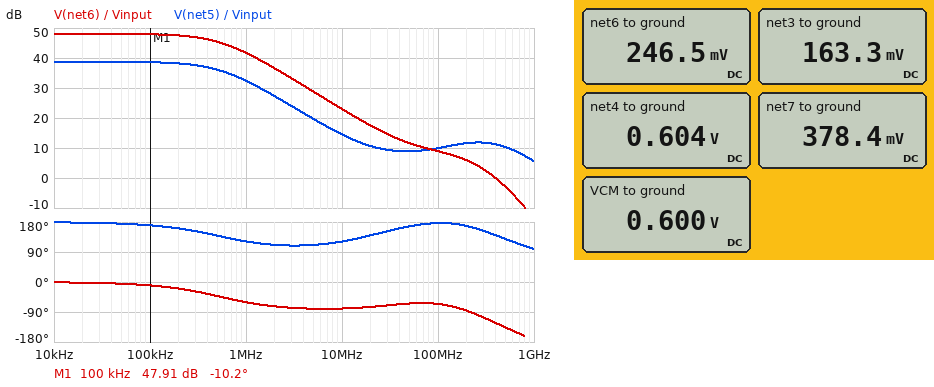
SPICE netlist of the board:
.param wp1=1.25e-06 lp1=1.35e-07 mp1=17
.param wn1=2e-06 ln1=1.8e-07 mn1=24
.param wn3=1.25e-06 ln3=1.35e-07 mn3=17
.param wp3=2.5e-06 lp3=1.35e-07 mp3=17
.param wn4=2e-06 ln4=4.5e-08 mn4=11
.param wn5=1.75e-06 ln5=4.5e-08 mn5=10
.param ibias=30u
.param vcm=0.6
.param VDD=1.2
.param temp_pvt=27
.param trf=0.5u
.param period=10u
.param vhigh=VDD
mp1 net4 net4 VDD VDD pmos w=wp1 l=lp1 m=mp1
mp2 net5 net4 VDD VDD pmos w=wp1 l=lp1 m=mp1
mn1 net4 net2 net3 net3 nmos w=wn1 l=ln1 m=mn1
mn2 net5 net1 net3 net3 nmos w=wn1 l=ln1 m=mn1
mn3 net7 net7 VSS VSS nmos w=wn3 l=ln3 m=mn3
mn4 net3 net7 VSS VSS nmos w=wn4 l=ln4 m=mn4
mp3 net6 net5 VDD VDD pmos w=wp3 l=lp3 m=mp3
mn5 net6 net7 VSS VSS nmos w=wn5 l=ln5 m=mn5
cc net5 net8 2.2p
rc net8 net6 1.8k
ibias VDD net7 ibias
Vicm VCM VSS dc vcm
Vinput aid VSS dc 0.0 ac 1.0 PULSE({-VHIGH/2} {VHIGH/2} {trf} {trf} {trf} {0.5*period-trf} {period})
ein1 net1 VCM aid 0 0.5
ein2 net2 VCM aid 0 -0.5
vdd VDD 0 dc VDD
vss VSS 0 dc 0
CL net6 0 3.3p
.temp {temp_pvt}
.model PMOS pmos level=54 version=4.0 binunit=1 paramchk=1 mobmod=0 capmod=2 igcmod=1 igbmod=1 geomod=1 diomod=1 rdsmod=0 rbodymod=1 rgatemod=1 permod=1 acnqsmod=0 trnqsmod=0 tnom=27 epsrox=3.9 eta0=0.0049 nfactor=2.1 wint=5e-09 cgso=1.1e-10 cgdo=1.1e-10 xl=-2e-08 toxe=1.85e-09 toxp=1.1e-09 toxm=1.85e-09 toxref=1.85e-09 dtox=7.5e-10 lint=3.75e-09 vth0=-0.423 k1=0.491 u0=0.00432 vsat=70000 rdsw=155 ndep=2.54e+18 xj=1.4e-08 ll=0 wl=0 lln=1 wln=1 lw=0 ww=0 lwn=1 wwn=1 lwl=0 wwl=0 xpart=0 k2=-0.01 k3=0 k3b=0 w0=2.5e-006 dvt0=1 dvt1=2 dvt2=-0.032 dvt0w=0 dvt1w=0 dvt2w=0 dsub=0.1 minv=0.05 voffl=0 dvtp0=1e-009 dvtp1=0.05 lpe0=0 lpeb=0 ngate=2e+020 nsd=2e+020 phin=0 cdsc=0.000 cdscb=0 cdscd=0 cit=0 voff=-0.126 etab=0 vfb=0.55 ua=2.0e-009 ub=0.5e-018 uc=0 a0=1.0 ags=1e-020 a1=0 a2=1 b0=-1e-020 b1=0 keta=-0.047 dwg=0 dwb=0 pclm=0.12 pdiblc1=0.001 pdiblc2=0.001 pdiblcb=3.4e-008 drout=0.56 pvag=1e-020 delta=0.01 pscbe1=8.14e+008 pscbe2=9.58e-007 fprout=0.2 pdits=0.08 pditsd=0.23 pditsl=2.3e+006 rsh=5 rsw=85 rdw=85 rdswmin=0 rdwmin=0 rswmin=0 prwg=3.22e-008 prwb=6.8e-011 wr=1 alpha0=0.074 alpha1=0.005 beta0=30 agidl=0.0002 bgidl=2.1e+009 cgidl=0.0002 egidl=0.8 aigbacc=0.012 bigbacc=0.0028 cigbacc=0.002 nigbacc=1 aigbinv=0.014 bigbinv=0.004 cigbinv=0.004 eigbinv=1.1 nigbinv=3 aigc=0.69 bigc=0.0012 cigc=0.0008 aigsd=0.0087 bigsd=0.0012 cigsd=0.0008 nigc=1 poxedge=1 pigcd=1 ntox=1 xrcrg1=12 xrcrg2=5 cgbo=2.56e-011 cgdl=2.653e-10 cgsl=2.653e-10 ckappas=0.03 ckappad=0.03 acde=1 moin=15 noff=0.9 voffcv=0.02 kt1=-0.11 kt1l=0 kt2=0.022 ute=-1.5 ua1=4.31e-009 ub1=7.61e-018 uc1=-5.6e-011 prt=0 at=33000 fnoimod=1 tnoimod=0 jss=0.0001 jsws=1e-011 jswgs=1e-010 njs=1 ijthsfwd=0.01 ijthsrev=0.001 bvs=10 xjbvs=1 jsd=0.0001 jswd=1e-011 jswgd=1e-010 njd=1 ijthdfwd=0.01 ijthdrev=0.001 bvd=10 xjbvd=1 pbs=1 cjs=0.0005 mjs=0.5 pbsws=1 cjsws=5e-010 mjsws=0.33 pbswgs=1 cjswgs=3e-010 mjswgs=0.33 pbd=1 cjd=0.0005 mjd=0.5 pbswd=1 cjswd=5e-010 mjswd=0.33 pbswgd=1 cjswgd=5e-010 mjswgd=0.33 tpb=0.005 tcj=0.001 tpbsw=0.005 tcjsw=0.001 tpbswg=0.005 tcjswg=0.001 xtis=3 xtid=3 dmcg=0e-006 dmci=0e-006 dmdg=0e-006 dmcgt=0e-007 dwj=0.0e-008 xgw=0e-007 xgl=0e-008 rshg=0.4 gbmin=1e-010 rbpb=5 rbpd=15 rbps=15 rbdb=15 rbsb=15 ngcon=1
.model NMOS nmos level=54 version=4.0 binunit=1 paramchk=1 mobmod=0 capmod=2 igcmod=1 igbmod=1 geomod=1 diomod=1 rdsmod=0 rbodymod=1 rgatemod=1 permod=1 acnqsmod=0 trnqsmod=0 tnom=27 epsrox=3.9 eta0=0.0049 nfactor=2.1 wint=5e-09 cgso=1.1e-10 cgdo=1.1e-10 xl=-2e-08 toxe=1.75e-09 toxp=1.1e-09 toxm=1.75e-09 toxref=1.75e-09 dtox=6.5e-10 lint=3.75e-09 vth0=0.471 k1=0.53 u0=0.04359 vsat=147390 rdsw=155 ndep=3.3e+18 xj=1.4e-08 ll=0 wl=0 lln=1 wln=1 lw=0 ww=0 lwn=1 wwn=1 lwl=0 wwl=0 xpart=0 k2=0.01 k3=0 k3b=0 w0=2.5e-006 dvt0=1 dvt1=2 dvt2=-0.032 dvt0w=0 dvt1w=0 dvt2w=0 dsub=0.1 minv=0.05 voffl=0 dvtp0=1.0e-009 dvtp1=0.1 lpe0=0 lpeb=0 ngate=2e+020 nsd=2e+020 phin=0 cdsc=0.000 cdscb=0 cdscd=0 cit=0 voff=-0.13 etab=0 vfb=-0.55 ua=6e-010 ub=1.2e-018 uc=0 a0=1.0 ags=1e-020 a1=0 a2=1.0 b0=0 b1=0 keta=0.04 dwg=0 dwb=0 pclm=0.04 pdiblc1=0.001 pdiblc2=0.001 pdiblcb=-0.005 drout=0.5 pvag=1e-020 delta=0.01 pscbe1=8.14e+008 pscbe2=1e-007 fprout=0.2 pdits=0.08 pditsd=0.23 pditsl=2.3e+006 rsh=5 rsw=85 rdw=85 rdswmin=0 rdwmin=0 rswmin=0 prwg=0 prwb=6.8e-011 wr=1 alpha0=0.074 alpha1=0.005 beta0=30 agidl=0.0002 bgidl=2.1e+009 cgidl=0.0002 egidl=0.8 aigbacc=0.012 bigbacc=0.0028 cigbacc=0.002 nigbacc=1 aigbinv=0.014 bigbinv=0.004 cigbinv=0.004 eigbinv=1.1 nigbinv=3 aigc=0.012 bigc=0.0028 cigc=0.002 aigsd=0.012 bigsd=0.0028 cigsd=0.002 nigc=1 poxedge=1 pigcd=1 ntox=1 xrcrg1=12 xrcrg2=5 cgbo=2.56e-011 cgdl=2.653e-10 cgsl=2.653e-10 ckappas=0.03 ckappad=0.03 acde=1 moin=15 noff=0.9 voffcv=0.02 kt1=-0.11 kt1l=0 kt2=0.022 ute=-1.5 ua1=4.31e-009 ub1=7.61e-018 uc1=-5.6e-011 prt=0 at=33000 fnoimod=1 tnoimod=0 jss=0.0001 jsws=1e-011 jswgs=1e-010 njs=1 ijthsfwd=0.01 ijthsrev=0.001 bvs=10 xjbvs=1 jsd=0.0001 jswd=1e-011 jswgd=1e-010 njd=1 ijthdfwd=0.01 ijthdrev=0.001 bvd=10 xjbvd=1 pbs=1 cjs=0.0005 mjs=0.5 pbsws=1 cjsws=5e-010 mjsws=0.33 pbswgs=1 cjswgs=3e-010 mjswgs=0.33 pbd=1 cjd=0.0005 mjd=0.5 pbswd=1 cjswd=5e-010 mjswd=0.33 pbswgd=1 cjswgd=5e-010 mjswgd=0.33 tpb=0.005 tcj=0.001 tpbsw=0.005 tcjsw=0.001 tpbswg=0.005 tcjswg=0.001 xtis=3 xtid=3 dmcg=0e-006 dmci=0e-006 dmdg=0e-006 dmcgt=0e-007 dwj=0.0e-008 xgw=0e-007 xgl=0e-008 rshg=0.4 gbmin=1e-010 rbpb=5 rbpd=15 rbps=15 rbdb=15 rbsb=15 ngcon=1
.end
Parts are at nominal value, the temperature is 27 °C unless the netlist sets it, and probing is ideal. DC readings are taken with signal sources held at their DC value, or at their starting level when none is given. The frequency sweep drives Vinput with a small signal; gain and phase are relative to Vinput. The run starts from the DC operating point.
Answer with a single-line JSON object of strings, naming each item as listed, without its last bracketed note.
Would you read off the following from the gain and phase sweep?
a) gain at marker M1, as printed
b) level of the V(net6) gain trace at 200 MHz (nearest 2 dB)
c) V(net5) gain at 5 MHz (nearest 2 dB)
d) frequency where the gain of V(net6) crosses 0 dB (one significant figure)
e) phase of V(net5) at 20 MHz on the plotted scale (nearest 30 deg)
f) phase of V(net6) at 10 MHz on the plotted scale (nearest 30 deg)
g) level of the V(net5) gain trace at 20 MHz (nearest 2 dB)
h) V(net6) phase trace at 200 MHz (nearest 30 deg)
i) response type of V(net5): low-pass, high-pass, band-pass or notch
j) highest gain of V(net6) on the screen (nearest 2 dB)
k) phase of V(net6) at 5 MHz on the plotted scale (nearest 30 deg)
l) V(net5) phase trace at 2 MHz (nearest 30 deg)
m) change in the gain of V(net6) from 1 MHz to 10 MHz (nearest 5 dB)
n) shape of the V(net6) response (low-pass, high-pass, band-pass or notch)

{"gain at marker M1, as printed": "47.91 dB", "level of the V(net6) gain trace at 200 MHz": "6 dB", "V(net5) gain at 5 MHz": "20 dB", "frequency where the gain of V(net6) crosses 0 dB": "400 MHz", "phase of V(net5) at 20 MHz on the plotted scale": "150 deg", "phase of V(net6) at 10 MHz on the plotted scale": "-90 deg", "level of the V(net5) gain trace at 20 MHz": "10 dB", "V(net6) phase trace at 200 MHz": "-90 deg", "response type of V(net5): low-pass, high-pass, band-pass or notch": "low-pass", "highest gain of V(net6) on the screen": "48 dB", "phase of V(net6) at 5 MHz on the plotted scale": "-90 deg", "V(net5) phase trace at 2 MHz": "120 deg", "change in the gain of V(net6) from 1 MHz to 10 MHz": "-20 dB", "shape of the V(net6) response": "low-pass"}
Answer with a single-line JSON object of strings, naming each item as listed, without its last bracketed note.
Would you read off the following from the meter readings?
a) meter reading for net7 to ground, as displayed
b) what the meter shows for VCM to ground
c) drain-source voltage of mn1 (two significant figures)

{"meter reading for net7 to ground, as displayed": "378.4 mV", "what the meter shows for VCM to ground": "0.600 V", "drain-source voltage of mn1": "440 mV"}
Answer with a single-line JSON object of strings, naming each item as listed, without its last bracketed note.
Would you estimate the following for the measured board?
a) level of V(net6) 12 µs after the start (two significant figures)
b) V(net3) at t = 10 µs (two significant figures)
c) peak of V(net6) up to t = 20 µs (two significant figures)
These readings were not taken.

{"level of V(net6) 12 µs after the start": "980 mV", "V(net3) at t = 10 µs": "360 mV", "peak of V(net6) up to t = 20 µs": "980 mV"}
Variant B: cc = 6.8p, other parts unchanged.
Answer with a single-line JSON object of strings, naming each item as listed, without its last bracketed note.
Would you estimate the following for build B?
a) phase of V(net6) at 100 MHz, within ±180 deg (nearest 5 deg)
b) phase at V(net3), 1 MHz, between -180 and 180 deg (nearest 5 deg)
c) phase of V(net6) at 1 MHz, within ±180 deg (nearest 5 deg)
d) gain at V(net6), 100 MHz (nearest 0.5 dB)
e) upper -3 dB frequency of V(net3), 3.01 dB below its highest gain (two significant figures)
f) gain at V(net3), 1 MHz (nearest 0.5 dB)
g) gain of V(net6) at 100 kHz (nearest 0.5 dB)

{"phase of V(net6) at 100 MHz, within ±180 deg": "-50 deg", "phase at V(net3), 1 MHz, between -180 and 180 deg": "110 deg", "phase of V(net6) at 1 MHz, within ±180 deg": "-75 deg", "gain at V(net6), 100 MHz": "8.5 dB", "upper -3 dB frequency of V(net3), 3.01 dB below its highest gain": "180 kHz", "gain at V(net3), 1 MHz": "-29.0 dB", "gain of V(net6) at 100 kHz": "47.0 dB"}
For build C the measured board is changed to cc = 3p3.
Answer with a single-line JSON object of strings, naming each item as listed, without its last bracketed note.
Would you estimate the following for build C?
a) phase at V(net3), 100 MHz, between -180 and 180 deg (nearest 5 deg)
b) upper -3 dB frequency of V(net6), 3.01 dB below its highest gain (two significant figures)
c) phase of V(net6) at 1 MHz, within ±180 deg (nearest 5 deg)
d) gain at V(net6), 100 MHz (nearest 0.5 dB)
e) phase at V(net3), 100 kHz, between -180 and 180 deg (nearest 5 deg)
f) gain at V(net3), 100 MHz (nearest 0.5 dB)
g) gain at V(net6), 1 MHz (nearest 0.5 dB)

{"phase at V(net3), 100 MHz, between -180 and 180 deg": "-150 deg", "upper -3 dB frequency of V(net6), 3.01 dB below its highest gain": "370 kHz", "phase of V(net6) at 1 MHz, within ±180 deg": "-70 deg", "gain at V(net6), 100 MHz": "8.5 dB", "phase at V(net3), 100 kHz, between -180 and 180 deg": "165 deg", "gain at V(net3), 100 MHz": "-32.5 dB", "gain at V(net6), 1 MHz": "39.0 dB"}
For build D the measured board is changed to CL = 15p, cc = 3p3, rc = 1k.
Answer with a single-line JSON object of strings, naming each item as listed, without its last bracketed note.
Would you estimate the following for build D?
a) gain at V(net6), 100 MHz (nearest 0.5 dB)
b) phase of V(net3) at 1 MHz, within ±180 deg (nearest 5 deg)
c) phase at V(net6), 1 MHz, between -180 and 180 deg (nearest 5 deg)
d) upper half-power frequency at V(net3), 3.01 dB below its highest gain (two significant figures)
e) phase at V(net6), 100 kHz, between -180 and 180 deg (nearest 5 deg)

{"gain at V(net6), 100 MHz": "-4.5 dB", "phase of V(net3) at 1 MHz, within ±180 deg": "120 deg", "phase at V(net6), 1 MHz, between -180 and 180 deg": "-70 deg", "upper half-power frequency at V(net3), 3.01 dB below its highest gain": "370 kHz", "phase at V(net6), 100 kHz, between -180 and 180 deg": "-15 deg"}
